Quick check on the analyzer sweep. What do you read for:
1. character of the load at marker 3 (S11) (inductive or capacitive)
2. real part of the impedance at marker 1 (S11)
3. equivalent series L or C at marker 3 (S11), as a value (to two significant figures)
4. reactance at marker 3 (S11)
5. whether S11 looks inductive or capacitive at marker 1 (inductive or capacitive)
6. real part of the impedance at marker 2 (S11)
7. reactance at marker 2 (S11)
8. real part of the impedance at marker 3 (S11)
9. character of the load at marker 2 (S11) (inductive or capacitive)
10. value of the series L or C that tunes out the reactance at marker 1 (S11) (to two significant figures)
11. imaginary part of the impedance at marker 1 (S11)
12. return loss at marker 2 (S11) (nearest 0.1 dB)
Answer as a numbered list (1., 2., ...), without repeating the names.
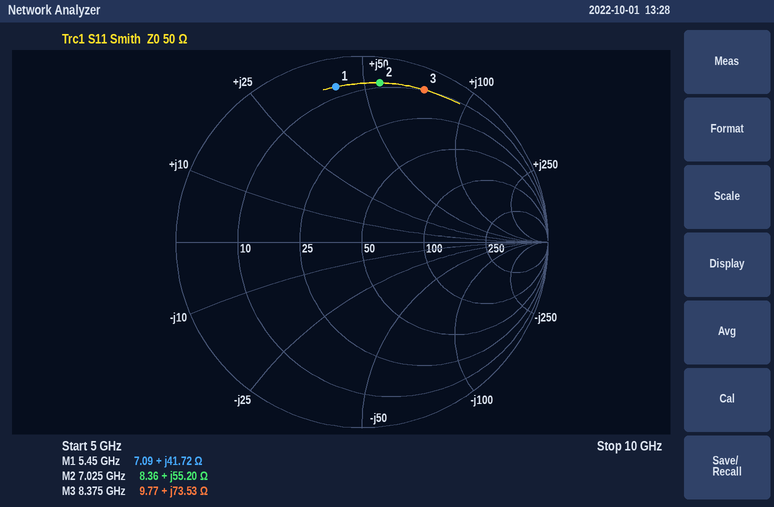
1. inductive
2. 7.09 Ω
3. 1.4 nH
4. +73.53 Ω
5. inductive
6. 8.36 Ω
7. +55.20 Ω
8. 9.77 Ω
9. inductive
10. 700 fF
11. +41.72 Ω
12. 1.3 dB
